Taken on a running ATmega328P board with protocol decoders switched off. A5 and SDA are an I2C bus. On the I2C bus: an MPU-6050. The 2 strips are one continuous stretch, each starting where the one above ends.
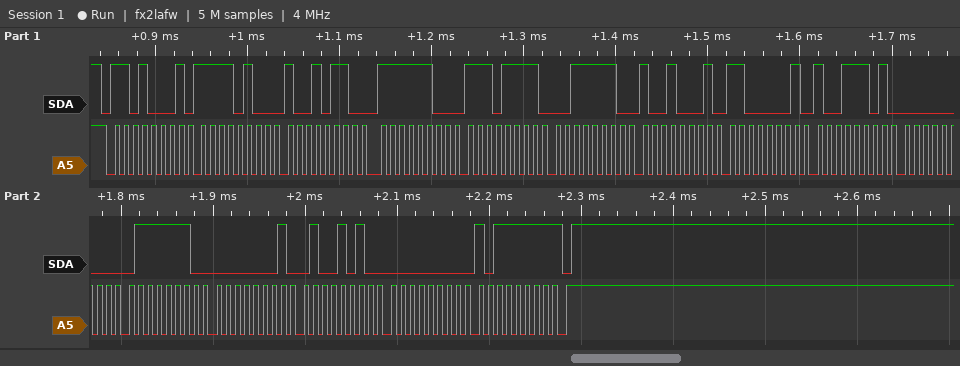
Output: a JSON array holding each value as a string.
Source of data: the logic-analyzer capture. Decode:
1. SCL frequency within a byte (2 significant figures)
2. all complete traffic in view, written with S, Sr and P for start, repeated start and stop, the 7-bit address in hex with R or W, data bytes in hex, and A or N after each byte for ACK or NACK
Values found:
["100 kHz", "S 68R A F4 A 96 A FC A EF A 3E A 91 A C1 A 9D A 00 A 7E A 01 A 4A A 00 A BF N P"]
